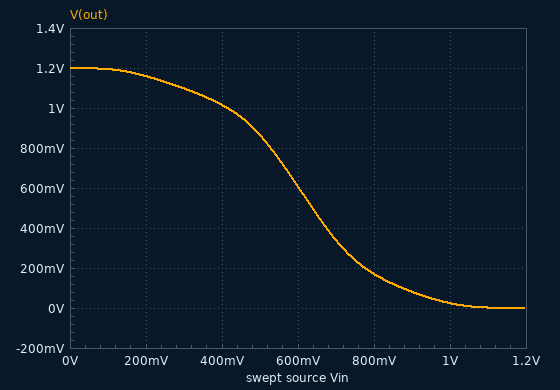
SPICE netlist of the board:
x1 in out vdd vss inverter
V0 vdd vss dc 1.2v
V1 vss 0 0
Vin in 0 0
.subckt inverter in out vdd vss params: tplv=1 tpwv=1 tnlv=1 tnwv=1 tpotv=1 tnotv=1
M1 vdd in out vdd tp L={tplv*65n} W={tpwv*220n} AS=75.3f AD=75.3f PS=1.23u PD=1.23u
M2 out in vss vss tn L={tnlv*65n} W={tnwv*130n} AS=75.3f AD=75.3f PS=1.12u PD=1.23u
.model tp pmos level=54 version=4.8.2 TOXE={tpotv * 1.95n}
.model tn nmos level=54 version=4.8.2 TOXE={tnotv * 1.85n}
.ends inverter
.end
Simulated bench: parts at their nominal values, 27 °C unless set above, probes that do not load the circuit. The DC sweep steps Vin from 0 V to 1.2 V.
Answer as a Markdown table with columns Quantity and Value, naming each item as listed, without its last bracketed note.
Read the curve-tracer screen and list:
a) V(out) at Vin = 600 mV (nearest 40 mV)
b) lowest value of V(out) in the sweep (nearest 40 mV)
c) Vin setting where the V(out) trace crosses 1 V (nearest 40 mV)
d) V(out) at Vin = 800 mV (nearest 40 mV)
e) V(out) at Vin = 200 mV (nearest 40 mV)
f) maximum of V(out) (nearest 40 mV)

| Quantity | Value |
|---|---|
| V(out) at Vin = 600 mV | 600 mV |
| lowest value of V(out) in the sweep | 0 V |
| Vin setting where the V(out) trace crosses 1 V | 400 mV |
| V(out) at Vin = 800 mV | 160 mV |
| V(out) at Vin = 200 mV | 1.16 V |
| maximum of V(out) | 1.20 V |
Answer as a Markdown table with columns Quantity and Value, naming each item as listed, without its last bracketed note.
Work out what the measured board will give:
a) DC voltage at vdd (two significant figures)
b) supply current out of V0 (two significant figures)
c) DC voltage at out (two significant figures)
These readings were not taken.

| Quantity | Value |
|---|---|
| DC voltage at vdd | 1.2 V |
| supply current out of V0 | 130 nA |
| DC voltage at out | 1.2 V |
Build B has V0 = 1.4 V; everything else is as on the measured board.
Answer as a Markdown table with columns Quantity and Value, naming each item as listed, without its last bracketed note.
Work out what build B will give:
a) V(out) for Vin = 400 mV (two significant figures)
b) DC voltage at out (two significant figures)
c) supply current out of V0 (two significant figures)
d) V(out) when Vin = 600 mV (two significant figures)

| Quantity | Value |
|---|---|
| V(out) for Vin = 400 mV | 1.2 V |
| DC voltage at out | 1.4 V |
| supply current out of V0 | 180 nA |
| V(out) when Vin = 600 mV | 990 mV |
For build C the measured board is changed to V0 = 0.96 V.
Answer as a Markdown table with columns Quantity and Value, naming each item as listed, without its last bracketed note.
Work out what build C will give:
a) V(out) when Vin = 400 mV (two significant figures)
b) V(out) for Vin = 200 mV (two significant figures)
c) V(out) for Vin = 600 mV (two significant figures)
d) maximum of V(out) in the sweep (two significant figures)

| Quantity | Value |
|---|---|
| V(out) when Vin = 400 mV | 680 mV |
| V(out) for Vin = 200 mV | 920 mV |
| V(out) for Vin = 600 mV | 150 mV |
| maximum of V(out) in the sweep | 960 mV |
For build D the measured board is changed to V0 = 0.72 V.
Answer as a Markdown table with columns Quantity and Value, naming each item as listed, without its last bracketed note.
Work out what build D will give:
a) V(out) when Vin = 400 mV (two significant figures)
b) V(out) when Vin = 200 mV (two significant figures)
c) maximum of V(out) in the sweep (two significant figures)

| Quantity | Value |
|---|---|
| V(out) when Vin = 400 mV | 160 mV |
| V(out) when Vin = 200 mV | 680 mV |
| maximum of V(out) in the sweep | 720 mV |
